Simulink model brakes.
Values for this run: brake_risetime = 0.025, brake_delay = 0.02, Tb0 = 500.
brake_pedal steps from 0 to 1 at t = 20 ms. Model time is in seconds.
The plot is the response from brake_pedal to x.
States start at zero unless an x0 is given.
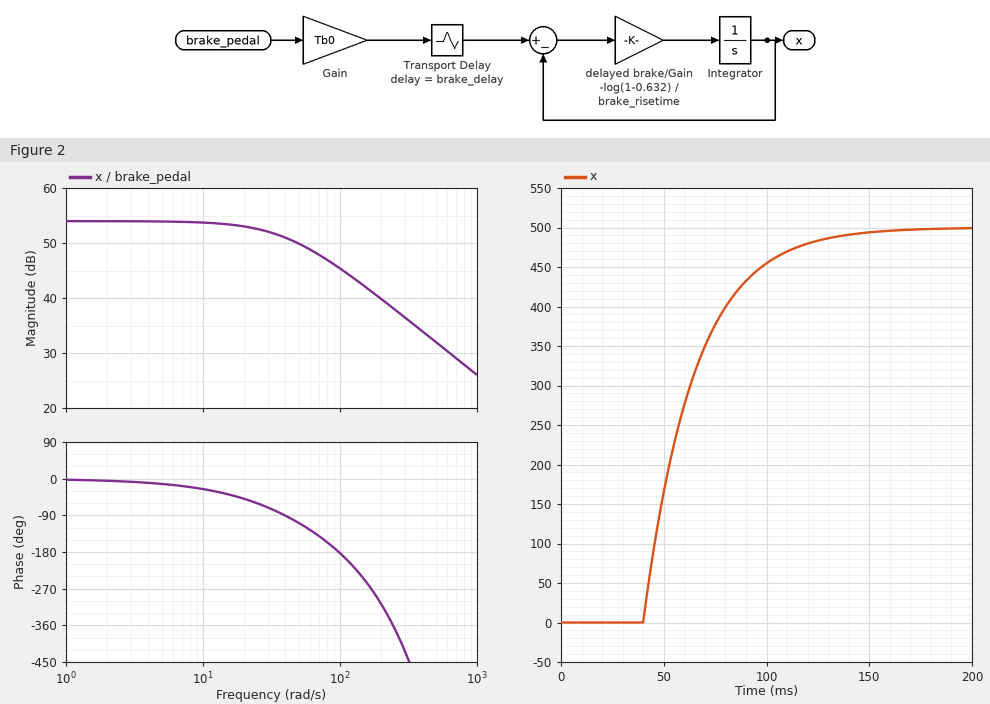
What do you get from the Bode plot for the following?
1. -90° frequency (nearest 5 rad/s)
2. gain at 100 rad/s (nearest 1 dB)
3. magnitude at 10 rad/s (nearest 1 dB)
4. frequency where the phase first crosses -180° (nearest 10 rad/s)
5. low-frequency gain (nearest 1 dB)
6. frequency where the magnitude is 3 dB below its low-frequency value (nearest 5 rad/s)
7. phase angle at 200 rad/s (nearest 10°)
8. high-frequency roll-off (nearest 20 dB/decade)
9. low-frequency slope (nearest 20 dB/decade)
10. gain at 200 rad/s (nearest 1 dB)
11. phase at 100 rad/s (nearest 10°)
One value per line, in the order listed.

40 rad/s
45 dB
54 dB
100 rad/s
54 dB
40 rad/s
-310°
-20 dB/decade
0 dB/decade
40 dB
-180°
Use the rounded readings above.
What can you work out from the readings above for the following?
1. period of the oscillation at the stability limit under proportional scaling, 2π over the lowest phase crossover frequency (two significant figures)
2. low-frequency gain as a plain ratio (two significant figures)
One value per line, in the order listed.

0.063 s
500
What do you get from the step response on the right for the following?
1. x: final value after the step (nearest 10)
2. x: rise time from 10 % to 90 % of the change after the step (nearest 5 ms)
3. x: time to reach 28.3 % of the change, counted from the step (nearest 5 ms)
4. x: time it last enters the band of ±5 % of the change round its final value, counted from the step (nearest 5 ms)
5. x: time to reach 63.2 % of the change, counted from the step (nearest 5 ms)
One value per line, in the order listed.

500
55 ms
30 ms
95 ms
45 ms
